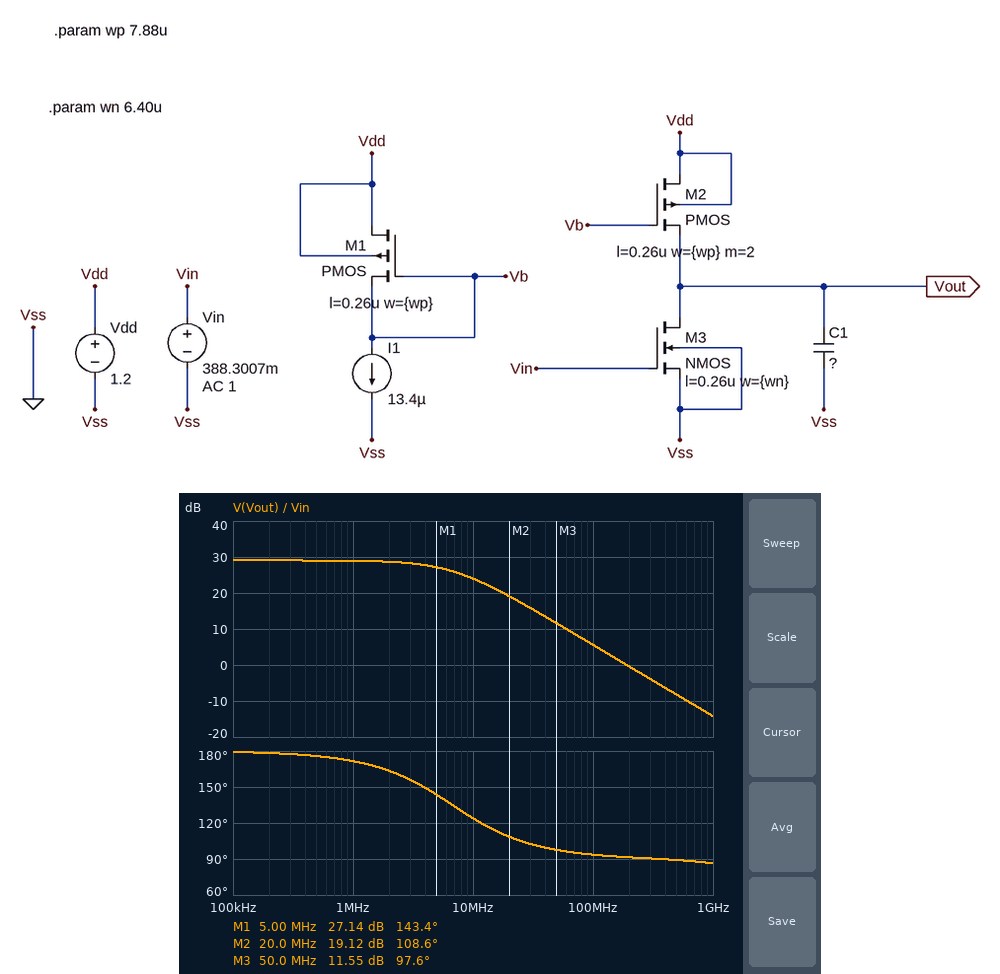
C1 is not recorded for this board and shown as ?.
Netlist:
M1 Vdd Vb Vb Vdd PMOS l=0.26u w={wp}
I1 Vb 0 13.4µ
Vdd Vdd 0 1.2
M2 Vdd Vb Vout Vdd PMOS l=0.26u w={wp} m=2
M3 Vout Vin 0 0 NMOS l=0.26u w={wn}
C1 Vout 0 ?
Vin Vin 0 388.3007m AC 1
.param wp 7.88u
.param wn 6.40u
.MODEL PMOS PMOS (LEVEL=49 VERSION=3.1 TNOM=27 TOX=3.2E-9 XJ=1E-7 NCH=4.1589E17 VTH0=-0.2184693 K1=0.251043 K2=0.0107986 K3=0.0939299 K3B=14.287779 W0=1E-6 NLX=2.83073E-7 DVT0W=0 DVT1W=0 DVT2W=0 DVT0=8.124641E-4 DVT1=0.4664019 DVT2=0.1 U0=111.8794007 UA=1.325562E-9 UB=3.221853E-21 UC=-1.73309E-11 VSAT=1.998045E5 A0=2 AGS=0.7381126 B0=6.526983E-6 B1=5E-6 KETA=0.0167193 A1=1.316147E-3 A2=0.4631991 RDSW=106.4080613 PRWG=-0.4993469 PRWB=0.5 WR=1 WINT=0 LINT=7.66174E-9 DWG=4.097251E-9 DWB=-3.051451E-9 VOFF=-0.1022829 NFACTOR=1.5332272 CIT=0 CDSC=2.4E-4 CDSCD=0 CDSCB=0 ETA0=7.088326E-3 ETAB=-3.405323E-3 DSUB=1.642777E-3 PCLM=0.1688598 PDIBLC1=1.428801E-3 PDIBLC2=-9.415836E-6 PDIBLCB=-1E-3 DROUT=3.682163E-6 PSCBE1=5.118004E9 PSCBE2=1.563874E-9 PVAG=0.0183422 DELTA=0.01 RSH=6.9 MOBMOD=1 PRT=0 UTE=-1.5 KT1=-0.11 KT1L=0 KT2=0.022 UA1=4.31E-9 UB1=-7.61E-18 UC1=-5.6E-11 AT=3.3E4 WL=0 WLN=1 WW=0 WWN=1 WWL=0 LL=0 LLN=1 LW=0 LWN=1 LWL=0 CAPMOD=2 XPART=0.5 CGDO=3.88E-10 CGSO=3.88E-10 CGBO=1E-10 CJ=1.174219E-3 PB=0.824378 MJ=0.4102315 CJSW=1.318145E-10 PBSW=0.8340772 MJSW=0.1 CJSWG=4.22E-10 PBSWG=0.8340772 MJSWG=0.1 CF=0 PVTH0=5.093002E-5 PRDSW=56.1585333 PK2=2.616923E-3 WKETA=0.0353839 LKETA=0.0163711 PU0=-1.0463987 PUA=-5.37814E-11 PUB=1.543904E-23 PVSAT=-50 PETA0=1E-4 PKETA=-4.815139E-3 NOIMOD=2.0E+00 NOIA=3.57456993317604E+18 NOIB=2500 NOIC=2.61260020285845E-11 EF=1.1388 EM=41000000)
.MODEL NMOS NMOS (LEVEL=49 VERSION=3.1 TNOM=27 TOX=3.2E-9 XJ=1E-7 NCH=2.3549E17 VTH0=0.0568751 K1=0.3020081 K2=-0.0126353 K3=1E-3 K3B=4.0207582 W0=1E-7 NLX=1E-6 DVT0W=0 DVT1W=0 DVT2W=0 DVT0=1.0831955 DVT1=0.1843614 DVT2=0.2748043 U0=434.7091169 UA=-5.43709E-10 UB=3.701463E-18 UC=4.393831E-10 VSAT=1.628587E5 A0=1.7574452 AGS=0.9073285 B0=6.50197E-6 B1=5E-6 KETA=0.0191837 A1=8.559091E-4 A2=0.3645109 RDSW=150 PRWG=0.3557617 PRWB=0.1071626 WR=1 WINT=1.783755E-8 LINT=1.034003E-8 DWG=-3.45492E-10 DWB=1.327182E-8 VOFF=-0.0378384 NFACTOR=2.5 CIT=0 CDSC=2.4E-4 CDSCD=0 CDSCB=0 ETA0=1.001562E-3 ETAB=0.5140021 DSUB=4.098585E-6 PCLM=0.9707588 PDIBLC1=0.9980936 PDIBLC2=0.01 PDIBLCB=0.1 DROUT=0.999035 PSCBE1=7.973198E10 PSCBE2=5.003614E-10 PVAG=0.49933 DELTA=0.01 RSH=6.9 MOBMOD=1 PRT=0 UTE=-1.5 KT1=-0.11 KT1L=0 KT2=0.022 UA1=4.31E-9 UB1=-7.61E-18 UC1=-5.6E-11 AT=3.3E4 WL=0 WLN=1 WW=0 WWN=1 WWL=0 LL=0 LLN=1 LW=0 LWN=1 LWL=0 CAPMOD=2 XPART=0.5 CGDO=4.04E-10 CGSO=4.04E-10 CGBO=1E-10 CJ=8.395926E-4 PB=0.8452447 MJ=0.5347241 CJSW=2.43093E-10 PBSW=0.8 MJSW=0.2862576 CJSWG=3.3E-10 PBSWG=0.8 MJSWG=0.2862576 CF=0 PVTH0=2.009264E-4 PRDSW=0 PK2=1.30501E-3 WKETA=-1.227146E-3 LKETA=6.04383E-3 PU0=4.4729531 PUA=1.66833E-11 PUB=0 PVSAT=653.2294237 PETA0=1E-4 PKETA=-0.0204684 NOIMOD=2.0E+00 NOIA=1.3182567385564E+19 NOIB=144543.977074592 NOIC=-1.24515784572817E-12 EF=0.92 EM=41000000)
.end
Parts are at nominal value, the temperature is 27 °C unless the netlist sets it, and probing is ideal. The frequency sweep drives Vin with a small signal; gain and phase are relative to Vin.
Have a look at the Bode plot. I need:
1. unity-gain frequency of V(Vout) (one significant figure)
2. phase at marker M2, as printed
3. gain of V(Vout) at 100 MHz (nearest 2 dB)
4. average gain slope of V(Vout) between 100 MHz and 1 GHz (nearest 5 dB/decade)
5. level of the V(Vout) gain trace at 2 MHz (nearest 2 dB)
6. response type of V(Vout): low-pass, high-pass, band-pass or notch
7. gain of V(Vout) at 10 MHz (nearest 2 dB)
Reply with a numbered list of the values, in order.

1. 200 MHz
2. 108.6 deg
3. 6 dB
4. -20 dB/decade
5. 28 dB
6. low-pass
7. 24 dB
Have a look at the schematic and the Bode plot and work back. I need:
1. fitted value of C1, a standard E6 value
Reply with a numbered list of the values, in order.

1. 470 fF
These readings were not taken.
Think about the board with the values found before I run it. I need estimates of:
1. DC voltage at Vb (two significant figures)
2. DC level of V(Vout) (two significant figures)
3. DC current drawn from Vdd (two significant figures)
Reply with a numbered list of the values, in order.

1. 800 mV
2. 610 mV
3. 42 µA
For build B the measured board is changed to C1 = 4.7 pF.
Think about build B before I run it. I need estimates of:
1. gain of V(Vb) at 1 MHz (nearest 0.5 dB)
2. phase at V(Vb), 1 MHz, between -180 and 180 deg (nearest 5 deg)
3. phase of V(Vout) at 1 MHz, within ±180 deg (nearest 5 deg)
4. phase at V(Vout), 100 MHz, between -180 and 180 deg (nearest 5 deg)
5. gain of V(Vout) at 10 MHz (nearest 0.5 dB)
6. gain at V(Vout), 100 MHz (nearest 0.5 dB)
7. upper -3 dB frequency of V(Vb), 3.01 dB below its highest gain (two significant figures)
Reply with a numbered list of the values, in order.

1. -52.0 dB
2. -145 deg
3. 125 deg
4. 90 deg
5. 6.0 dB
6. -14.0 dB
7. 620 MHz
